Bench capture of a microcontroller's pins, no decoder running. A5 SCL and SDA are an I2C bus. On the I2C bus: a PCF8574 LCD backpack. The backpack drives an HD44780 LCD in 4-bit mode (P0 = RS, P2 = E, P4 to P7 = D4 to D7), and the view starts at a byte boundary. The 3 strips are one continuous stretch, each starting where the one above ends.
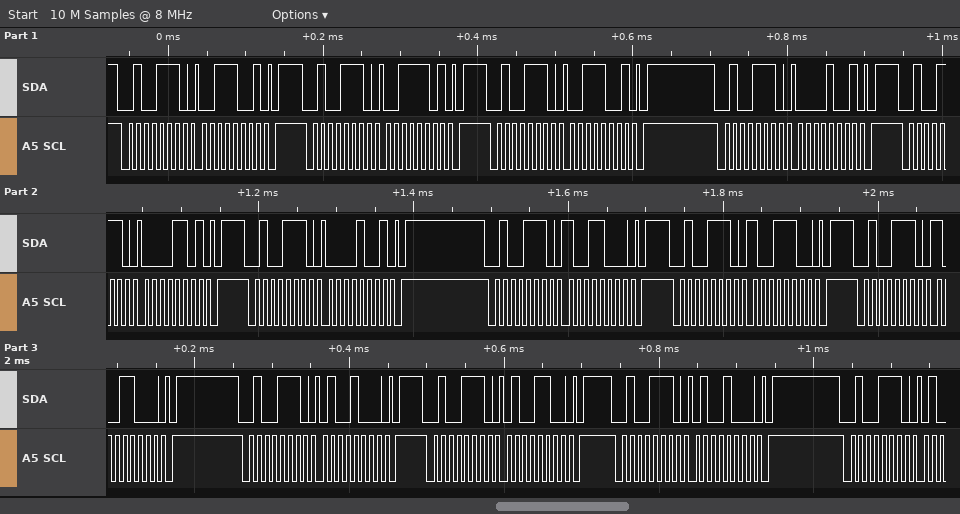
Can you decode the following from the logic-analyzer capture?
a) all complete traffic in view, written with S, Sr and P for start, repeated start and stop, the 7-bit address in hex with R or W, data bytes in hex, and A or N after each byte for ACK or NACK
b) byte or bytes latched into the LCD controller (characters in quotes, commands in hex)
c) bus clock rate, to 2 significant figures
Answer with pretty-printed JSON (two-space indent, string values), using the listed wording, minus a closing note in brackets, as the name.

{
  "all complete traffic in view, written with S, Sr and P for start, repeated start and stop, the 7-bit address in hex with R or W, data bytes in hex, and A or N after each byte for ACK or NACK": "S 27W A 39 A P S 27W A 3D A P S 27W A 39 A P S 27W A 09 A P S 27W A 0D A P S 27W A 09 A P S 27W A 98 A P S 27W A 9C A P S 27W A 98 A P S 27W A 48 A P S 27W A 4C A P S 27W A 48 A P S 27W A",
  "byte or bytes latched into the LCD controller": "'0' 0x94",
  "bus clock rate, to 2 significant figures": "100 kHz"
}
